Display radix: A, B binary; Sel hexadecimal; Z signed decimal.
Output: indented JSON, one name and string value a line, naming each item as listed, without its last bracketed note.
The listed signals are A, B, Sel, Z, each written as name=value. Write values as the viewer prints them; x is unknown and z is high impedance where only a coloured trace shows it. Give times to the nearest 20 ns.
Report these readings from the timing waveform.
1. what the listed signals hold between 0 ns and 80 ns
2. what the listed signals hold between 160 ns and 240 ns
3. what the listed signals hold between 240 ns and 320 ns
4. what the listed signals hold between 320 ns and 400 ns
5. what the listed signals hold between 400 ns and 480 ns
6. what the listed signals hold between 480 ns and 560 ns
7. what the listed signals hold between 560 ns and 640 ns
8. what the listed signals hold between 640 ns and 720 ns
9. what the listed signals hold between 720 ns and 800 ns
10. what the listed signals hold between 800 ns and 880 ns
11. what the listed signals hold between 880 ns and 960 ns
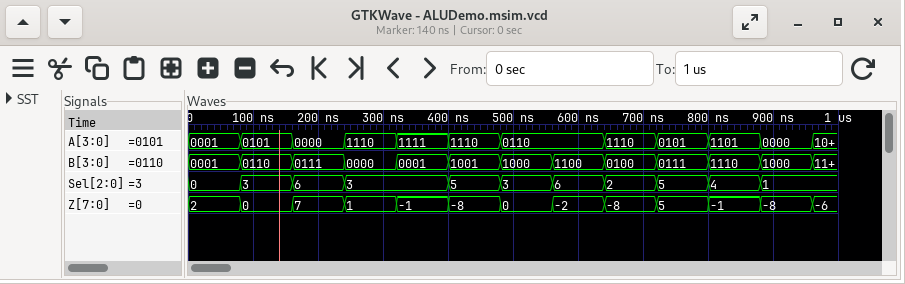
{
  "what the listed signals hold between 0 ns and 80 ns": "A=0001, B=0001, Sel=0, Z=2",
  "what the listed signals hold between 160 ns and 240 ns": "A=0000, B=0111, Sel=6, Z=7",
  "what the listed signals hold between 240 ns and 320 ns": "A=1110, B=0000, Sel=3, Z=1",
  "what the listed signals hold between 320 ns and 400 ns": "A=1111, B=0001, Sel=3, Z=-1",
  "what the listed signals hold between 400 ns and 480 ns": "A=1110, B=1001, Sel=5, Z=-8",
  "what the listed signals hold between 480 ns and 560 ns": "A=0110, B=1000, Sel=3, Z=0",
  "what the listed signals hold between 560 ns and 640 ns": "A=0110, B=1100, Sel=6, Z=-2",
  "what the listed signals hold between 640 ns and 720 ns": "A=1110, B=0100, Sel=2, Z=-8",
  "what the listed signals hold between 720 ns and 800 ns": "A=0101, B=0111, Sel=5, Z=5",
  "what the listed signals hold between 800 ns and 880 ns": "A=1101, B=1110, Sel=4, Z=-1",
  "what the listed signals hold between 880 ns and 960 ns": "A=0000, B=1000, Sel=1, Z=-8"
}
